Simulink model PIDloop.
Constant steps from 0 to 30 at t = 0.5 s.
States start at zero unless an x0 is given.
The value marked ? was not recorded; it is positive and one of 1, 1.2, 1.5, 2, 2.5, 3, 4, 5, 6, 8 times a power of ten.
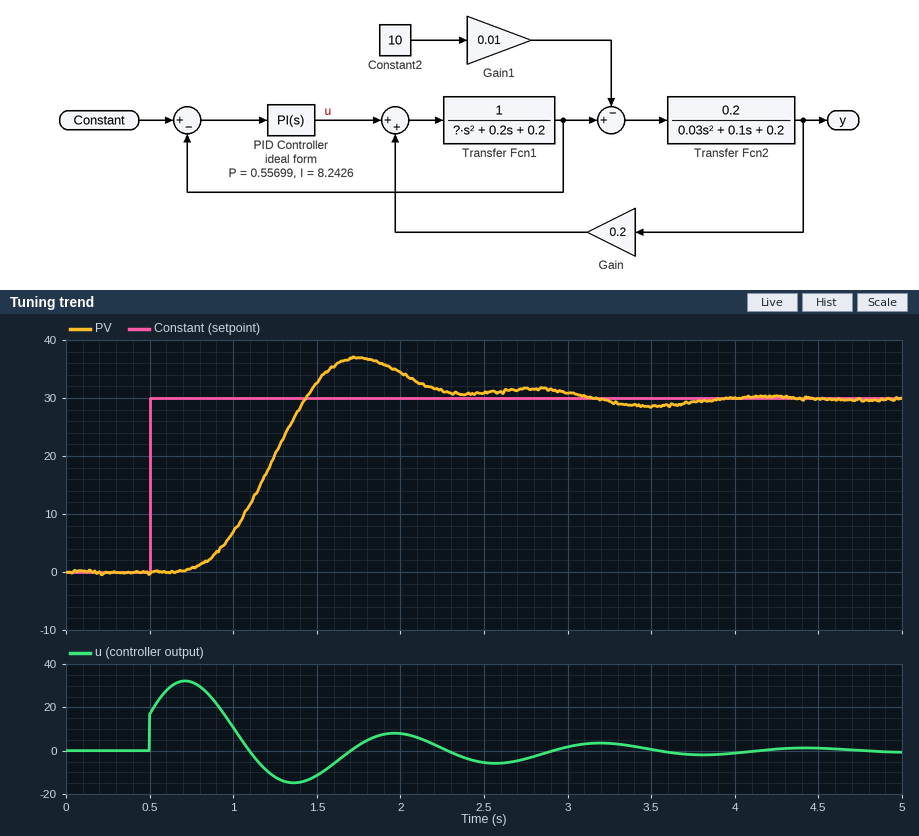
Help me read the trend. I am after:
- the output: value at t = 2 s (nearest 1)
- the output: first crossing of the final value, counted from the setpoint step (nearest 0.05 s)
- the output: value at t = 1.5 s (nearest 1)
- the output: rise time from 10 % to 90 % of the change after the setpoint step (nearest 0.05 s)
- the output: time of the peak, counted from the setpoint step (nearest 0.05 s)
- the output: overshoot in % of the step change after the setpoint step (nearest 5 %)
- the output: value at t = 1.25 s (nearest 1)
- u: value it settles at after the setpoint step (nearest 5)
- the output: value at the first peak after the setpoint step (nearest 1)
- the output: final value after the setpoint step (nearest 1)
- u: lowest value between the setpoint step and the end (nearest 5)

34
0.95 s
33
0.50 s
1.25 s
25 %
20
0
37
30
-15
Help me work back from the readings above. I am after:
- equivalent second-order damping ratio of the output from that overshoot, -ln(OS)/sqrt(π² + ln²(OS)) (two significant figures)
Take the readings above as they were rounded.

0.40
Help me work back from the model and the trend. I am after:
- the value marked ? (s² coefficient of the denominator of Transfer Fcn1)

0.02
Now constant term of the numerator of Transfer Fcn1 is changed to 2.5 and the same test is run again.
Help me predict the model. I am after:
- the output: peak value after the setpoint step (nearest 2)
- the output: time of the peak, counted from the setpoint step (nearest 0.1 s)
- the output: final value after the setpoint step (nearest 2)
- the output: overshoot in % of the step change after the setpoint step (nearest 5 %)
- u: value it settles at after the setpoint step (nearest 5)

34
1.5 s
30
15 %
-5
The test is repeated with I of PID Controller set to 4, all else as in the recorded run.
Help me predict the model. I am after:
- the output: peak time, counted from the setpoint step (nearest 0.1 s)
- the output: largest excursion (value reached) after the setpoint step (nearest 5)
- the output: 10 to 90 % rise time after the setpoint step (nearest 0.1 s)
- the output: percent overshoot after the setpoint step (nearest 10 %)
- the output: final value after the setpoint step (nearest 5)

1.6 s
40
0.6 s
30 %
30
